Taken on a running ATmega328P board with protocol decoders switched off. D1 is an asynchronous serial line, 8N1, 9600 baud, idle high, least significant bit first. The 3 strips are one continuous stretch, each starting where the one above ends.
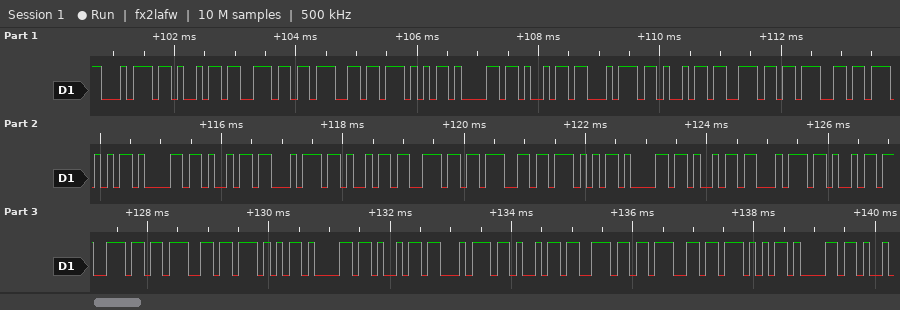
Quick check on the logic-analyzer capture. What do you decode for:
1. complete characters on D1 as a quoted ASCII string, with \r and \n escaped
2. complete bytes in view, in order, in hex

"tingWaitingWaitingWaitingWaitingWa"
0x74 0x69 0x6E 0x67 0x57 0x61 0x69 0x74 0x69 0x6E 0x67 0x57 0x61 0x69 0x74 0x69 0x6E 0x67 0x57 0x61 0x69 0x74 0x69 0x6E 0x67 0x57 0x61 0x69 0x74 0x69 0x6E 0x67 0x57 0x61
